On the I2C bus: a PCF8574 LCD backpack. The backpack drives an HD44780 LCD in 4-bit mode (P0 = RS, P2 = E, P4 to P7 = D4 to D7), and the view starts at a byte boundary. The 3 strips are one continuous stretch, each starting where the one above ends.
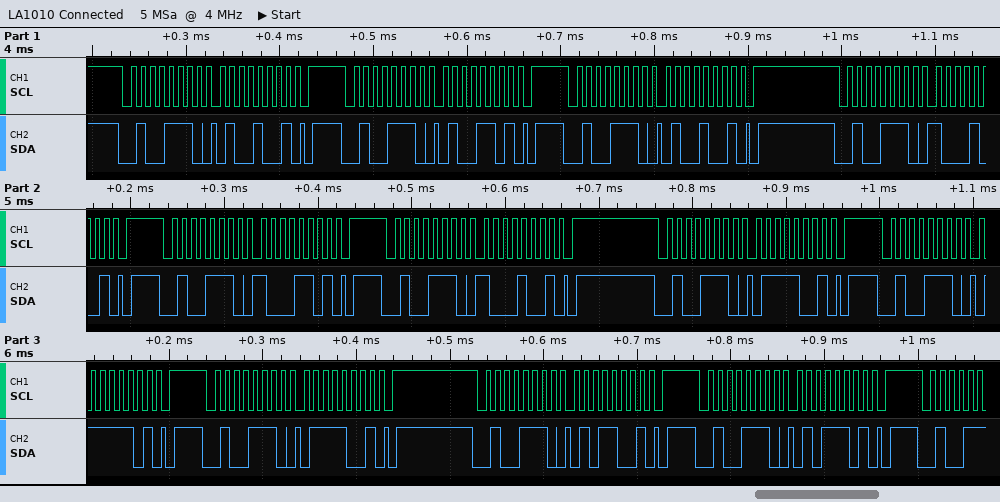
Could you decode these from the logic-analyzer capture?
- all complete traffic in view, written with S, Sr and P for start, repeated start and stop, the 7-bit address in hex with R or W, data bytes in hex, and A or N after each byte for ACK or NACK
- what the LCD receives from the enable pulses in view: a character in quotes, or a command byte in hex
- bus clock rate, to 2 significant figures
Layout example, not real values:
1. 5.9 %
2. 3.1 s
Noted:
1. S 27W A 49 A P S 27W A 4D A P S 27W A 49 A P S 27W A 89 A P S 27W A 8D A P S 27W A 89 A P S 27W A 79 A P S 27W A 7D A P S 27W A 79 A P S 27W A 59 A P S 27W A 5D A P
2. 'H'
3. 100 kHz
